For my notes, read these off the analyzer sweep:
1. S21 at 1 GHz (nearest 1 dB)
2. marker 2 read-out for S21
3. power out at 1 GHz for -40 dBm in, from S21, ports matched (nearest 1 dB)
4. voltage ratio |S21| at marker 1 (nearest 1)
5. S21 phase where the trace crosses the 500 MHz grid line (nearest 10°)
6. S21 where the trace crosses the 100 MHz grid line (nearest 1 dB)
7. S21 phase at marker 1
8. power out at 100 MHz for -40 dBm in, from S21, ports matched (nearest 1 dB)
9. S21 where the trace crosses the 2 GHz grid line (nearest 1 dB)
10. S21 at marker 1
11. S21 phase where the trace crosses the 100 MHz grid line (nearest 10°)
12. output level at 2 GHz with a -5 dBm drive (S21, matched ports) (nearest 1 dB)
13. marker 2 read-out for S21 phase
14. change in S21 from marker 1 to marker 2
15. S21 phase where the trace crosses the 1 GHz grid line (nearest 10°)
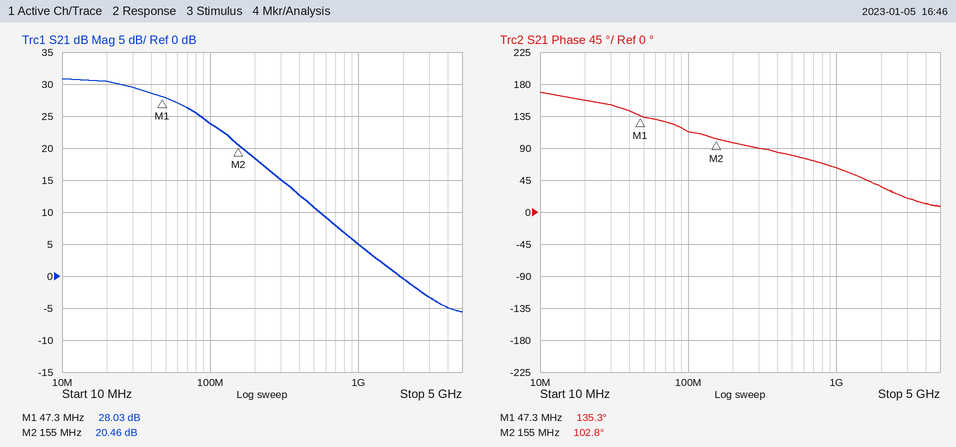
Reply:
5 dB
20.46 dB
-35 dBm
25
80°
24 dB
135.3°
-16 dBm
0 dB
28.03 dB
110°
-5 dBm
102.8°
-7.57 dB
60°
